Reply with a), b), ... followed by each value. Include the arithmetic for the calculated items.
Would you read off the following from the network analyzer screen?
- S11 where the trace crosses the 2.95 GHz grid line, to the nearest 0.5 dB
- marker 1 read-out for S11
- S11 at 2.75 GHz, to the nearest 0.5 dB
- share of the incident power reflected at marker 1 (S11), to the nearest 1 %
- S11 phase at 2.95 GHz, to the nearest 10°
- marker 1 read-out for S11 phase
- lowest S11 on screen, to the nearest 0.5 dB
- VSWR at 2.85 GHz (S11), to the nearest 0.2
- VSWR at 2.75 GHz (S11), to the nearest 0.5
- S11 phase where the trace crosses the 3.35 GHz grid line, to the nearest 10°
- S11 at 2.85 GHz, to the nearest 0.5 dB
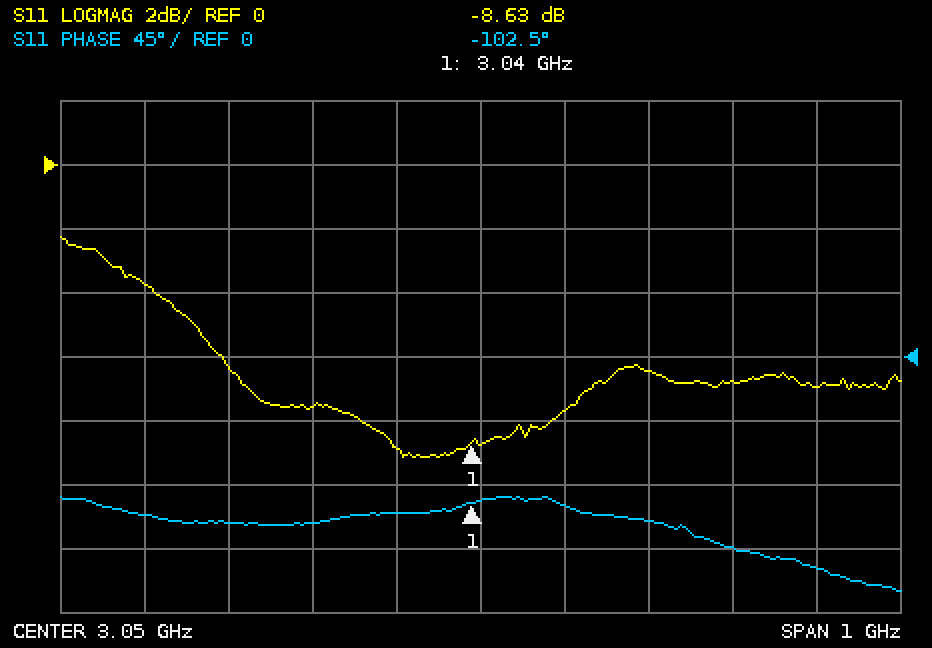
a) -9.0 dB
b) -8.63 dB
c) -6.5 dB
d) 10^(-8.63/10) ≈ 14 %
e) -110°
f) -102.5°
g) -9.0 dB
h) |Γ| = 10^(-7.5/20) = 0.4217; VSWR = (1 + 0.4217)/(1 − 0.4217) ≈ 2.46, so 2.4 to the nearest 0.2
i) |Γ| = 10^(-6.5/20) = 0.4732; VSWR = (1 + 0.4732)/(1 − 0.4732) ≈ 2.80, so 3.0 to the nearest 0.5
j) -130°
k) -7.5 dB
